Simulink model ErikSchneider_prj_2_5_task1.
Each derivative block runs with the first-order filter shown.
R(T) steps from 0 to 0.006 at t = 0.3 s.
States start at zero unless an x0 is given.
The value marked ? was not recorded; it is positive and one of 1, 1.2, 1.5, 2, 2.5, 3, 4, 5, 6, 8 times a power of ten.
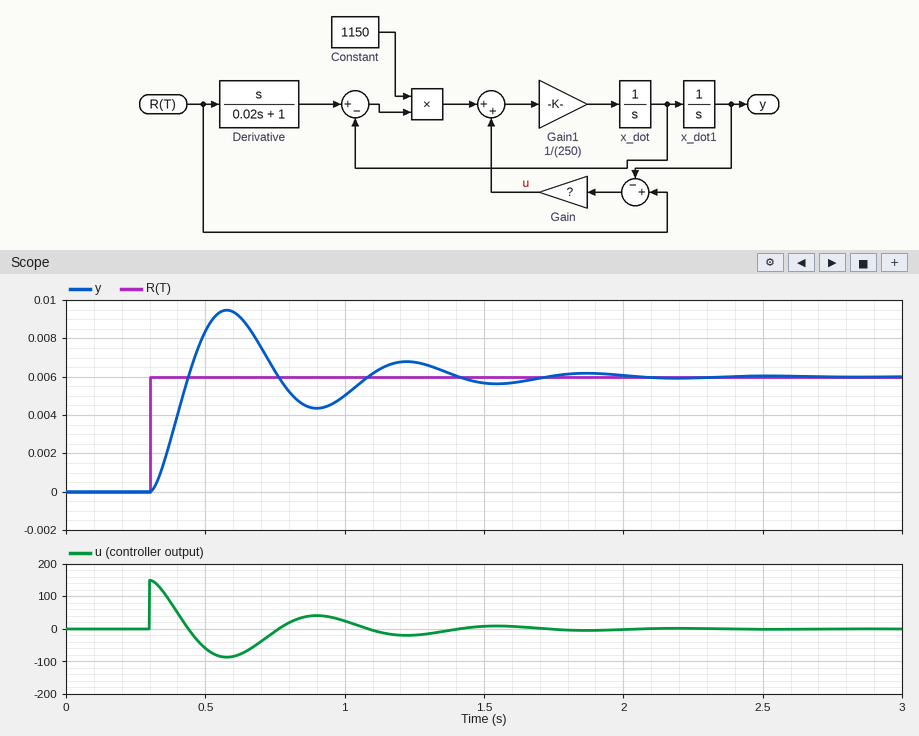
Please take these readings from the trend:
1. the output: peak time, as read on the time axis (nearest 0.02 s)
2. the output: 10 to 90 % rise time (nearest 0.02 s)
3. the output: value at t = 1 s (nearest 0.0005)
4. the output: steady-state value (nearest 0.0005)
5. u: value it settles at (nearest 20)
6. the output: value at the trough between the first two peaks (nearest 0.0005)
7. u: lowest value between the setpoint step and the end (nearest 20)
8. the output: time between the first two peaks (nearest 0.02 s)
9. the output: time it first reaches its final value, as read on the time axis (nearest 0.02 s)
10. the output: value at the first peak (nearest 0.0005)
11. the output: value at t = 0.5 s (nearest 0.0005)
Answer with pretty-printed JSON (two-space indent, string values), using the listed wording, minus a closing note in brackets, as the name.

{
  "the output: peak time, as read on the time axis": "0.58 s",
  "the output: 10 to 90 % rise time": "0.10 s",
  "the output: value at t = 1 s": "0.0050",
  "the output: steady-state value": "0.0060",
  "u: value it settles at": "0",
  "the output: value at the trough between the first two peaks": "0.0045",
  "u: lowest value between the setpoint step and the end": "-80",
  "the output: time between the first two peaks": "0.64 s",
  "the output: time it first reaches its final value, as read on the time axis": "0.44 s",
  "the output: value at the first peak": "0.0095",
  "the output: value at t = 0.5 s": "0.0085"
}
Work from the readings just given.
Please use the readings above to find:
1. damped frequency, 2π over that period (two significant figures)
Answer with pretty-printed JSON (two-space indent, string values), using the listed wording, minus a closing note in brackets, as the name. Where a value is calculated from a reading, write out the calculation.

{
  "damped frequency, 2π over that period": "2π / 0.64 = 9.8 rad/s"
}
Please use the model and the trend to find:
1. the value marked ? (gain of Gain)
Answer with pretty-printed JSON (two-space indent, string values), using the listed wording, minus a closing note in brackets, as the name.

{
  "the value marked ?": "25000"
}
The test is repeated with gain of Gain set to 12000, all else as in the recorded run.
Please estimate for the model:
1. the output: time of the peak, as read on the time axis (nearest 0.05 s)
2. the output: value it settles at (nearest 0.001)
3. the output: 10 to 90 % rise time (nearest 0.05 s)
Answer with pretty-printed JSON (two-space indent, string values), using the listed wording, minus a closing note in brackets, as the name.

{
  "the output: time of the peak, as read on the time axis": "0.70 s",
  "the output: value it settles at": "0.006",
  "the output: 10 to 90 % rise time": "0.15 s"
}
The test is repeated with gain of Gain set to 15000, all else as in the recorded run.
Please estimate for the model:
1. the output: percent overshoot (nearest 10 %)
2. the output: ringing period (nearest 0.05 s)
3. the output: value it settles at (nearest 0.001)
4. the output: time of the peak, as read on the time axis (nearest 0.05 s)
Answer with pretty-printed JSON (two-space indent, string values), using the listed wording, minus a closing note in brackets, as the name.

{
  "the output: percent overshoot": "50 %",
  "the output: ringing period": "0.85 s",
  "the output: value it settles at": "0.006",
  "the output: time of the peak, as read on the time axis": "0.65 s"
}
